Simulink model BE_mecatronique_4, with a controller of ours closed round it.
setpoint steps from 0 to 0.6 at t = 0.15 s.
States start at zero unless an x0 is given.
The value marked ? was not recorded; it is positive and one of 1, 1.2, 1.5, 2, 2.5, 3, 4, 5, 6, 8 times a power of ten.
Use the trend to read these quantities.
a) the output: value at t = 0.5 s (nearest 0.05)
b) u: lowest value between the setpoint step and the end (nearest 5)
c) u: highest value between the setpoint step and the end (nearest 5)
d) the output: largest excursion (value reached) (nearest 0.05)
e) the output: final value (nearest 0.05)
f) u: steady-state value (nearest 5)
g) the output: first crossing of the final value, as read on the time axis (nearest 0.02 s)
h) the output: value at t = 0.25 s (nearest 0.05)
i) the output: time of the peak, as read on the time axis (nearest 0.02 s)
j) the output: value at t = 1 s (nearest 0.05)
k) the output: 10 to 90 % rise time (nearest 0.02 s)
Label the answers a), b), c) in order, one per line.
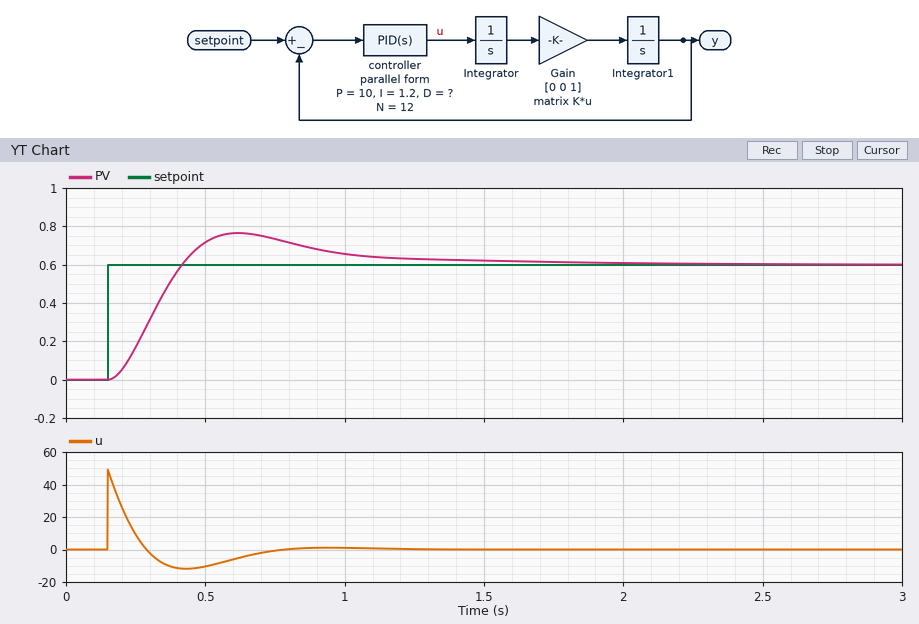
a) 0.70
b) -10
c) 50
d) 0.75
e) 0.60
f) 0
g) 0.42 s
h) 0.15
i) 0.62 s
j) 0.65
k) 0.18 s
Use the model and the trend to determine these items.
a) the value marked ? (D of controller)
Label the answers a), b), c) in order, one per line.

a) 6
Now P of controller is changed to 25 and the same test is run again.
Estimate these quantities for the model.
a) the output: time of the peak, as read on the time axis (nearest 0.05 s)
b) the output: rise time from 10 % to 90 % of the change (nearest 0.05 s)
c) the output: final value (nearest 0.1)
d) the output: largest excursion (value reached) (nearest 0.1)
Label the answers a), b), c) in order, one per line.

a) 0.55 s
b) 0.15 s
c) 0.6
d) 0.9
